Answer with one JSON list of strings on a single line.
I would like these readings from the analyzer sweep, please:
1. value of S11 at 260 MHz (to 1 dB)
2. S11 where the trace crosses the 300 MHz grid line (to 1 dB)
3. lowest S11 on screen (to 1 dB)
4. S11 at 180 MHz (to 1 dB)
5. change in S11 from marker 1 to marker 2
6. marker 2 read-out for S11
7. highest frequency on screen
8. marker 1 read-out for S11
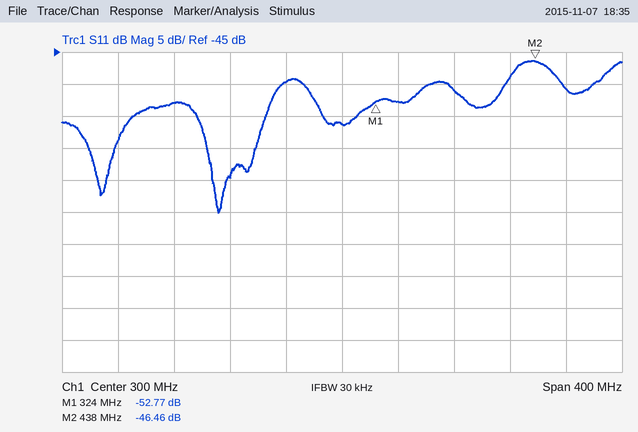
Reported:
["-50 dB", "-56 dB", "-70 dB", "-53 dB", "6.31 dB", "-46.46 dB", "500 MHz", "-52.77 dB"]
